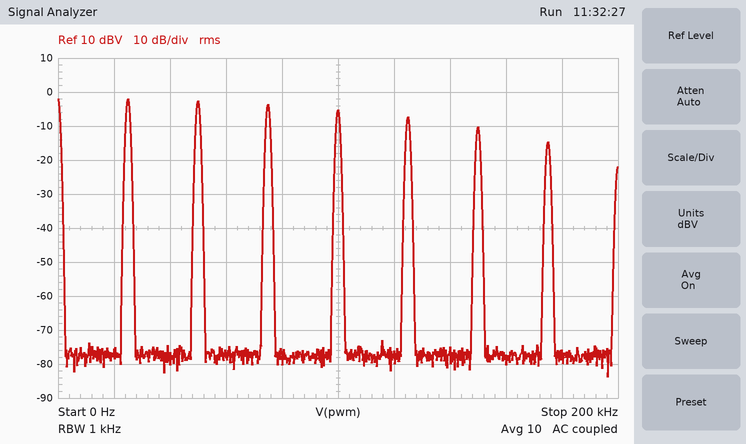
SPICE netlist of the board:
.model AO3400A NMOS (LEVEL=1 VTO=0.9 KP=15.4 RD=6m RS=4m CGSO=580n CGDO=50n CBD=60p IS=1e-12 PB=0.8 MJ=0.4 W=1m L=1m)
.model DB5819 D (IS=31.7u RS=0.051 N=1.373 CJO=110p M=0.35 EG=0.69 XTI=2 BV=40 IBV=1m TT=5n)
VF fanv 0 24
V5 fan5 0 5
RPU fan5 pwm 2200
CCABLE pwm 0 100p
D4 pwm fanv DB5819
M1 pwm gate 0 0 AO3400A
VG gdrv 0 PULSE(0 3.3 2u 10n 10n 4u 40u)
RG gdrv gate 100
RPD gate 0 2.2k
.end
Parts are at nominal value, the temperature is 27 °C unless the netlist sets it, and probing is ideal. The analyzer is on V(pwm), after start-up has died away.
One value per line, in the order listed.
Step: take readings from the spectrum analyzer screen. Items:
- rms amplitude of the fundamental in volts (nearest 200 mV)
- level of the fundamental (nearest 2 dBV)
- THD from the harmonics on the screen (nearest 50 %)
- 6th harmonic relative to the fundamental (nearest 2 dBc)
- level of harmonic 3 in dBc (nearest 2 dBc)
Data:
800 mV
-2 dBV
150 %
-8 dBc
-2 dBc
